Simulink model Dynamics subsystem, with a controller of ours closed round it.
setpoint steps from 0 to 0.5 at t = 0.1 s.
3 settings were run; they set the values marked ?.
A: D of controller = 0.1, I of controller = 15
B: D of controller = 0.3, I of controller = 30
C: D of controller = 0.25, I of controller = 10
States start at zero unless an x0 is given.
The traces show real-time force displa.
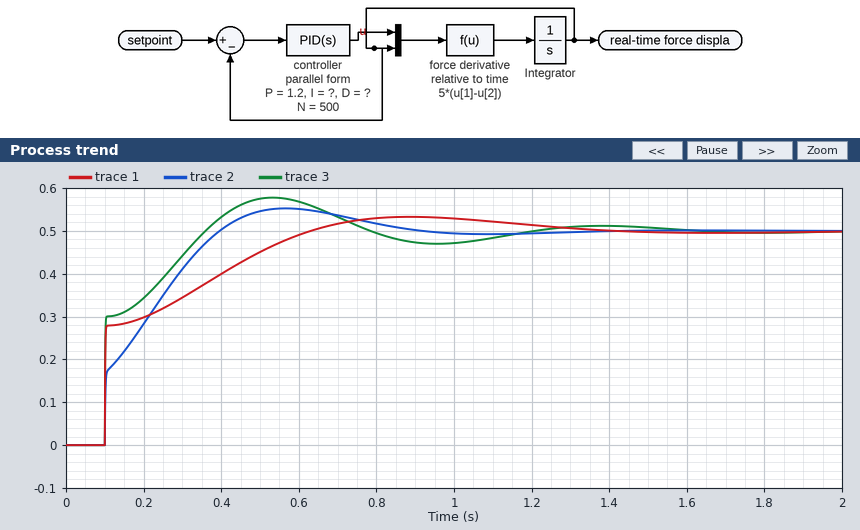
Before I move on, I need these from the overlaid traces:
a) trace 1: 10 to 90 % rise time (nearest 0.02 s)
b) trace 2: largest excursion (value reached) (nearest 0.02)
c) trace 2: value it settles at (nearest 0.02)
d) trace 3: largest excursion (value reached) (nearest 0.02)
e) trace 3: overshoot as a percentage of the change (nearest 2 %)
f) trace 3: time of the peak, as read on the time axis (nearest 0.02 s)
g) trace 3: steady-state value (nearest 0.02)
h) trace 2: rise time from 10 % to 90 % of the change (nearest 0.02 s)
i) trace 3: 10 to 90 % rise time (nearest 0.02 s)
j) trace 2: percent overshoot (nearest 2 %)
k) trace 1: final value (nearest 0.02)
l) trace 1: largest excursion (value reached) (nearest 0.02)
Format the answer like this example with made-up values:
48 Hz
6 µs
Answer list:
0.40 s
0.56
0.50
0.58
16 %
0.54 s
0.50
0.24 s
0.20 s
10 %
0.50
0.54
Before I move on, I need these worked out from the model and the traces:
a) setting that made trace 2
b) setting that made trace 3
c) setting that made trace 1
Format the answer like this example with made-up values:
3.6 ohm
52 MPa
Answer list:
A
B
C
